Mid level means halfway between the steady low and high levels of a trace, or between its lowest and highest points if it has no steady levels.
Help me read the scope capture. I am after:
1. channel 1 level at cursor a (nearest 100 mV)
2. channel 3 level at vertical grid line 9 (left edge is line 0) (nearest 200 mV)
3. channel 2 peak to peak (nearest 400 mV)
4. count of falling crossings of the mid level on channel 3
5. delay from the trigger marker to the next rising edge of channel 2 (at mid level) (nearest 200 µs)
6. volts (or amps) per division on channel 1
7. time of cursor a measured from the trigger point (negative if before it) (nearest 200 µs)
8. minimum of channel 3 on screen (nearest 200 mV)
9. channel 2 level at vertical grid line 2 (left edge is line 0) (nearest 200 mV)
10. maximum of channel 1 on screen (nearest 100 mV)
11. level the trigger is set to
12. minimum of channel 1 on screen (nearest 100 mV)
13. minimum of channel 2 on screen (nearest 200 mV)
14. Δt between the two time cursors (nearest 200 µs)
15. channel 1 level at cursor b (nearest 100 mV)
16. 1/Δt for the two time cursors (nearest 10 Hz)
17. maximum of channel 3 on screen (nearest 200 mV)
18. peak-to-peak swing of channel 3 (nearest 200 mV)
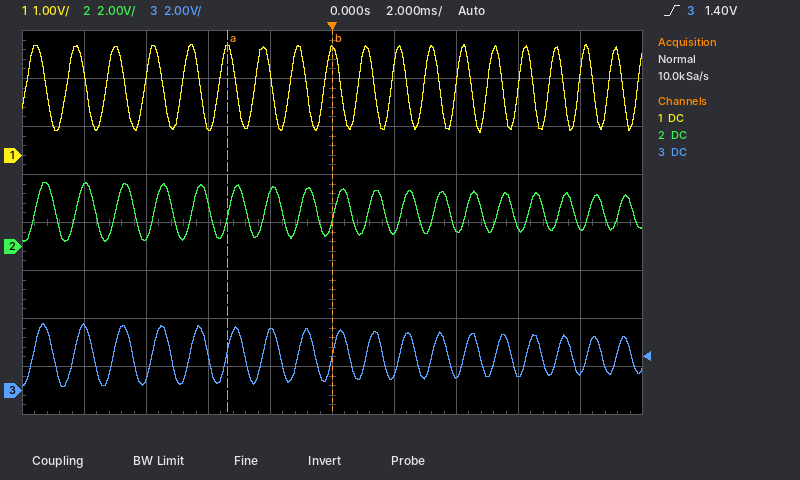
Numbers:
2.2 V
800 mV
2.4 V
18
1.2 ms
1 V
-3.4 ms
200 mV
400 mV
2.3 V
1.40 V
500 mV
200 mV
3.4 ms
2.2 V
290 Hz
2.8 V
2.6 V
